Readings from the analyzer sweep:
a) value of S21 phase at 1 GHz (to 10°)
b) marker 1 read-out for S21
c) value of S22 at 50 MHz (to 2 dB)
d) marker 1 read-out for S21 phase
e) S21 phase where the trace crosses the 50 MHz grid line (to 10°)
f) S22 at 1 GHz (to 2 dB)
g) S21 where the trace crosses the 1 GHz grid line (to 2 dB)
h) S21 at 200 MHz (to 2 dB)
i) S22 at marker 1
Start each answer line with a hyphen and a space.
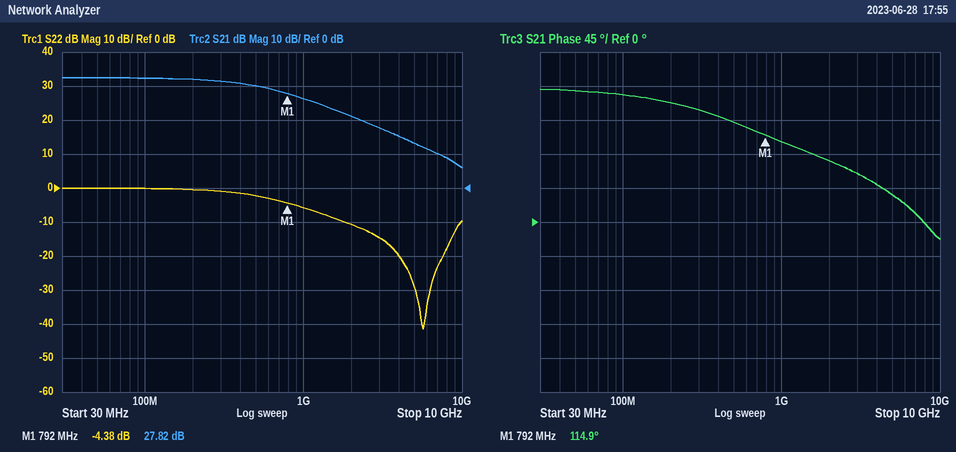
- 110°
- 27.82 dB
- 0 dB
- 114.9°
- 170°
- -6 dB
- 26 dB
- 32 dB
- -4.38 dB
